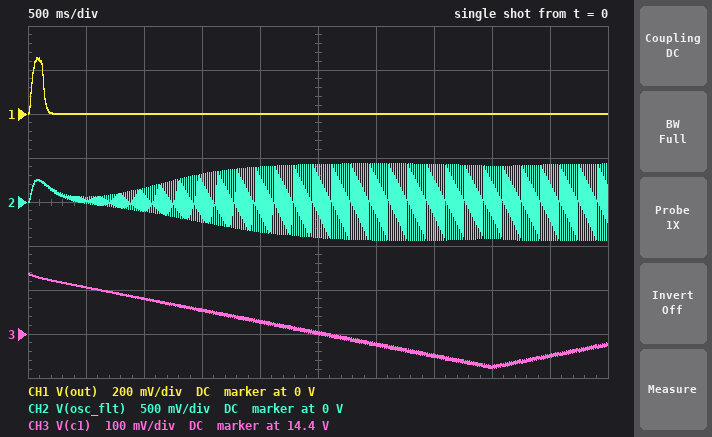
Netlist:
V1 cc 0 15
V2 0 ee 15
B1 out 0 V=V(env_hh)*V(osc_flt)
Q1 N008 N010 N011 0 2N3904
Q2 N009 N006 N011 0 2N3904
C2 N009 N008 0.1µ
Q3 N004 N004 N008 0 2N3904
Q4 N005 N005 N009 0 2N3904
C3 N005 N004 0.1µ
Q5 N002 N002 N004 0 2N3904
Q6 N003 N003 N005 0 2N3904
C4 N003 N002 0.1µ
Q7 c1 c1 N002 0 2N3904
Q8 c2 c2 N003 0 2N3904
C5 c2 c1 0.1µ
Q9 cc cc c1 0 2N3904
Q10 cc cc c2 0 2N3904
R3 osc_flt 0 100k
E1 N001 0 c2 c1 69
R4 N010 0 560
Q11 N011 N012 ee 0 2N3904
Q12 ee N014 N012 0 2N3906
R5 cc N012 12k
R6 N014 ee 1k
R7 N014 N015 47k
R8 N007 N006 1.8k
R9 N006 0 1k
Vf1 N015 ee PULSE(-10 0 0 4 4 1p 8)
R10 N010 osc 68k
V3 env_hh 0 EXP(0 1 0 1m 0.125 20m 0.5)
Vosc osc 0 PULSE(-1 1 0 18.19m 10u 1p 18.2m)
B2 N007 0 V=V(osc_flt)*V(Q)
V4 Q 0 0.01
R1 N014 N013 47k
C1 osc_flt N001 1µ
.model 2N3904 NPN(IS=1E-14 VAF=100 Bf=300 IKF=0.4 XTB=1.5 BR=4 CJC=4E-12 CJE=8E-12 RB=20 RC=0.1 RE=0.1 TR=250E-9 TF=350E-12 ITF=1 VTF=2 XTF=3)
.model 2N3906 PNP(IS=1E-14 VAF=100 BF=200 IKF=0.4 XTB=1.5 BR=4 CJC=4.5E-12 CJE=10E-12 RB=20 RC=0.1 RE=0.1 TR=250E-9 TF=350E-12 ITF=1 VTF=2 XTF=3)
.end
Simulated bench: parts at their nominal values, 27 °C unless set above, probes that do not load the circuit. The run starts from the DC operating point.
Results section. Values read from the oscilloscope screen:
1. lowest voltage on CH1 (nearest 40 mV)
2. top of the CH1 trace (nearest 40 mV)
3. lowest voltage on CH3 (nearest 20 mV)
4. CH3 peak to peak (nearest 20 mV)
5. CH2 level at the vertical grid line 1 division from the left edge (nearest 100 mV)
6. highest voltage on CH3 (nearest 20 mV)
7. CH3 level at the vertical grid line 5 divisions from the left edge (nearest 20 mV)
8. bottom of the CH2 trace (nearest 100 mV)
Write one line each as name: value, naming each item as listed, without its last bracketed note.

lowest voltage on CH1: 0 V
top of the CH1 trace: 240 mV
lowest voltage on CH3: 14.32 V
CH3 peak to peak: 220 mV
CH2 level at the vertical grid line 1 division from the left edge: 0 V
highest voltage on CH3: 14.54 V
CH3 level at the vertical grid line 5 divisions from the left edge: 14.40 V
bottom of the CH2 trace: -400 mV
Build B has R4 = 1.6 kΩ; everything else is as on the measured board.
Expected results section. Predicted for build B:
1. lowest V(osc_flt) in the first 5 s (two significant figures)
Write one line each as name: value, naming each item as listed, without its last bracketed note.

lowest V(osc_flt) in the first 5 s: -1.2 V
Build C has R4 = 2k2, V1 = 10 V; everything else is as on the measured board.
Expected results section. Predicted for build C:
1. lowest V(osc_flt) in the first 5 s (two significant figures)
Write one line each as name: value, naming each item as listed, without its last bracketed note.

lowest V(osc_flt) in the first 5 s: -1.6 V
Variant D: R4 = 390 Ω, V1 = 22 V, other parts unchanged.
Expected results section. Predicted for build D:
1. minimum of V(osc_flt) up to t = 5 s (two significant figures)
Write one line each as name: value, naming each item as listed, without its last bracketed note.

minimum of V(osc_flt) up to t = 5 s: -310 mV
